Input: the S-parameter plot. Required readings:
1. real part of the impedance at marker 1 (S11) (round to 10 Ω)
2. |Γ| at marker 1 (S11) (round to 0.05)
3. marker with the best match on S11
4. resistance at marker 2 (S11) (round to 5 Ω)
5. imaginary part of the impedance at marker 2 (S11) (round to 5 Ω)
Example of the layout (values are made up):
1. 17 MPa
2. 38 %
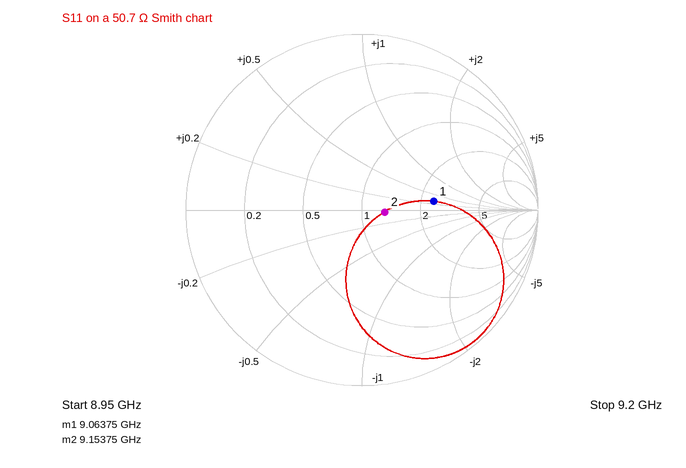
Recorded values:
1. 120 Ω
2. 0.40
3. marker 2
4. 65 Ω
5. 0 Ω
